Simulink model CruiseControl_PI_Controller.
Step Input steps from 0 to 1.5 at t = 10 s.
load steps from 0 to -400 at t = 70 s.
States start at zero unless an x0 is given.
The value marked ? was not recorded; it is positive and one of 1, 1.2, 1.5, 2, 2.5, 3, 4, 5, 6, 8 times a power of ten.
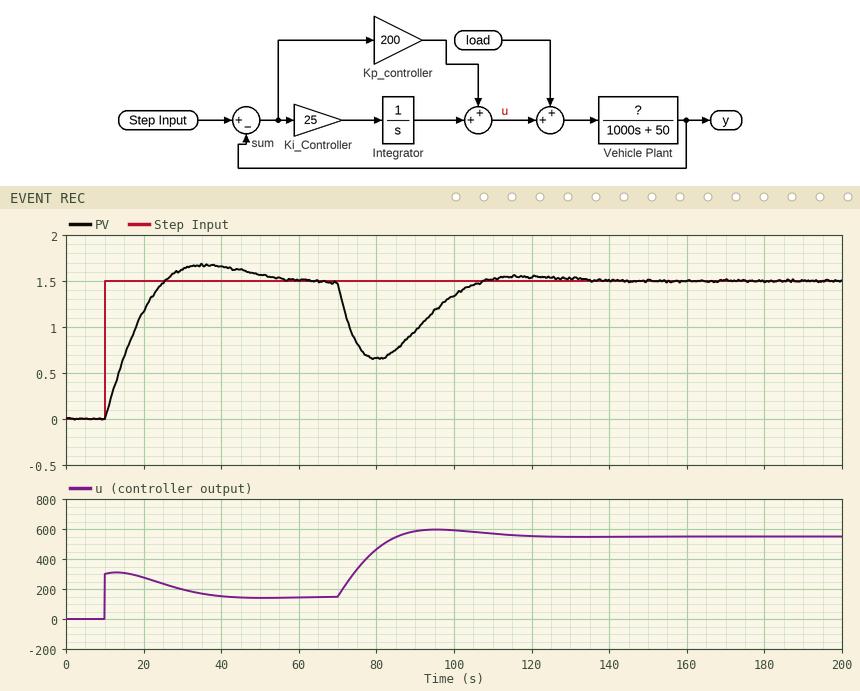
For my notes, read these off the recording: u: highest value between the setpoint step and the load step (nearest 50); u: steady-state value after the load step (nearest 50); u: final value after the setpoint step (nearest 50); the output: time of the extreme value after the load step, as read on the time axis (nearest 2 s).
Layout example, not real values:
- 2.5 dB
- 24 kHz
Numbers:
- 300
- 550
- 150
- 80 s
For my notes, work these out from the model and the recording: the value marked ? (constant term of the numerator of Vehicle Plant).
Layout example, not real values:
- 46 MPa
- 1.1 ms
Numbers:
- 0.5
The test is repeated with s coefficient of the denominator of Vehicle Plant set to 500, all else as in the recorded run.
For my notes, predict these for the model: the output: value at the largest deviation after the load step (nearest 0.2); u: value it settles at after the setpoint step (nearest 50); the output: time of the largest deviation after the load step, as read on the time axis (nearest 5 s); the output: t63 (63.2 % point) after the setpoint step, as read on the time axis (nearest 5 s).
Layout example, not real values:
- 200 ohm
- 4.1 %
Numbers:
- 0.6
- 150
- 75 s
- 15 s
